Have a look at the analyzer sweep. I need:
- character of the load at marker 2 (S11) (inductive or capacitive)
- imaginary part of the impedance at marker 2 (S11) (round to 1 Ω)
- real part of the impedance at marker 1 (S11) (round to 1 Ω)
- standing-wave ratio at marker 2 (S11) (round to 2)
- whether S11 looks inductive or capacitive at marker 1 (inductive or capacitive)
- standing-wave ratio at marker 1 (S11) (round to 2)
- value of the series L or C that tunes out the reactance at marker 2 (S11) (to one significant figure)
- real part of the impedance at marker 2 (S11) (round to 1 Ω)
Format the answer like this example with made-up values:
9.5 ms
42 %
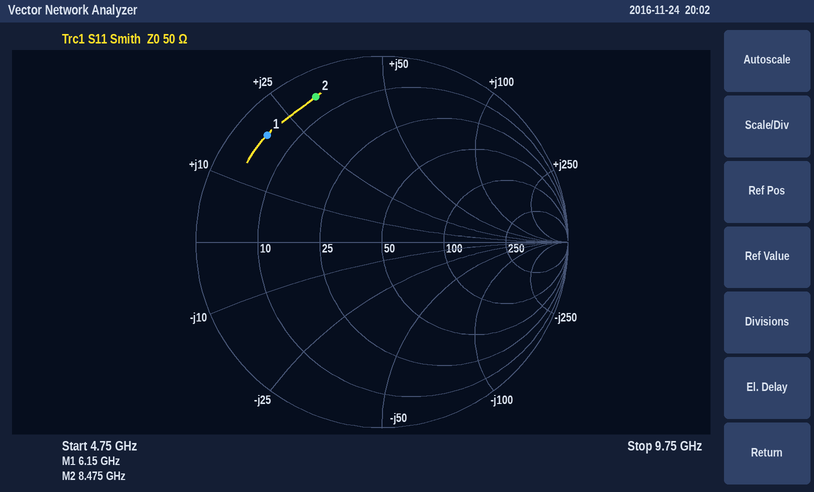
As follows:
inductive
+32 Ω
5 Ω
14
inductive
12
600 fF
5 Ω
